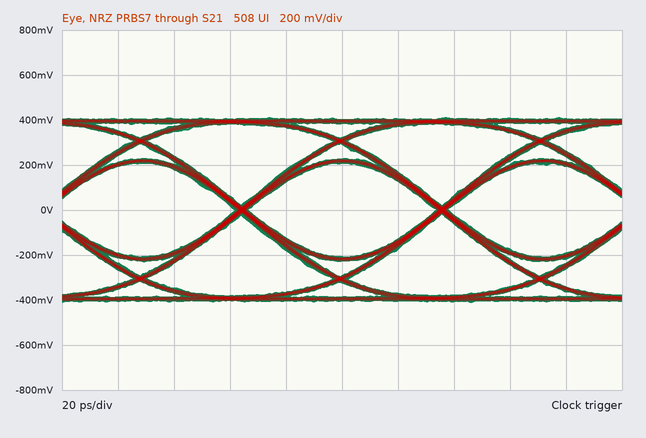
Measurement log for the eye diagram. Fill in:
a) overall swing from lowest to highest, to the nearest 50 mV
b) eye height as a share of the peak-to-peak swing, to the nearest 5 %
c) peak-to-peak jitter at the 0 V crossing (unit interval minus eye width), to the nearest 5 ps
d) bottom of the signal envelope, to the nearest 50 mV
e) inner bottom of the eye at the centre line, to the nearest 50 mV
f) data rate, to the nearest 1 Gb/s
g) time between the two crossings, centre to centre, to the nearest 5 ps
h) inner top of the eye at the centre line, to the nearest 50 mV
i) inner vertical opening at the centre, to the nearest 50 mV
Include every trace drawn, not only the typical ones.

800 mV
50 %
5 ps
-400 mV
-200 mV
14 Gb/s
70 ps
200 mV
400 mV
